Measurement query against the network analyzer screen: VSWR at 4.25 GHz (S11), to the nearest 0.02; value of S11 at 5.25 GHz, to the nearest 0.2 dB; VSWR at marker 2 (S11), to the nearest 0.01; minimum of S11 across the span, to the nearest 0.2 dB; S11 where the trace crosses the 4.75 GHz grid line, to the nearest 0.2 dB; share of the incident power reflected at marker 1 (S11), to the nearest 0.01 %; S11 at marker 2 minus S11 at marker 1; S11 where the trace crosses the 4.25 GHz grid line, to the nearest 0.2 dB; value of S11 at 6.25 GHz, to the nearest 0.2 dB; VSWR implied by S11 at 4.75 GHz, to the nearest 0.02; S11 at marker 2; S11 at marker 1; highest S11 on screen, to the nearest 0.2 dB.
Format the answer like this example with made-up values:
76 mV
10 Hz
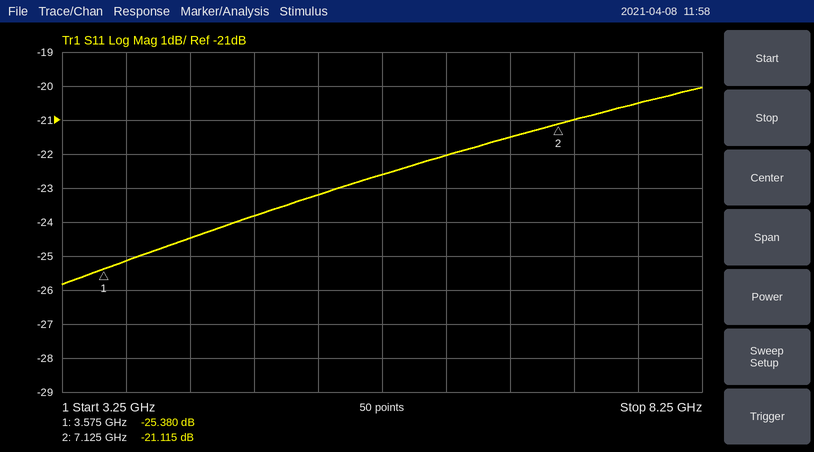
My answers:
1.12
-23.2 dB
1.19
-25.8 dB
-23.8 dB
0.29 %
4.265 dB
-24.4 dB
-22.0 dB
1.14
-21.115 dB
-25.380 dB
-20.0 dB
